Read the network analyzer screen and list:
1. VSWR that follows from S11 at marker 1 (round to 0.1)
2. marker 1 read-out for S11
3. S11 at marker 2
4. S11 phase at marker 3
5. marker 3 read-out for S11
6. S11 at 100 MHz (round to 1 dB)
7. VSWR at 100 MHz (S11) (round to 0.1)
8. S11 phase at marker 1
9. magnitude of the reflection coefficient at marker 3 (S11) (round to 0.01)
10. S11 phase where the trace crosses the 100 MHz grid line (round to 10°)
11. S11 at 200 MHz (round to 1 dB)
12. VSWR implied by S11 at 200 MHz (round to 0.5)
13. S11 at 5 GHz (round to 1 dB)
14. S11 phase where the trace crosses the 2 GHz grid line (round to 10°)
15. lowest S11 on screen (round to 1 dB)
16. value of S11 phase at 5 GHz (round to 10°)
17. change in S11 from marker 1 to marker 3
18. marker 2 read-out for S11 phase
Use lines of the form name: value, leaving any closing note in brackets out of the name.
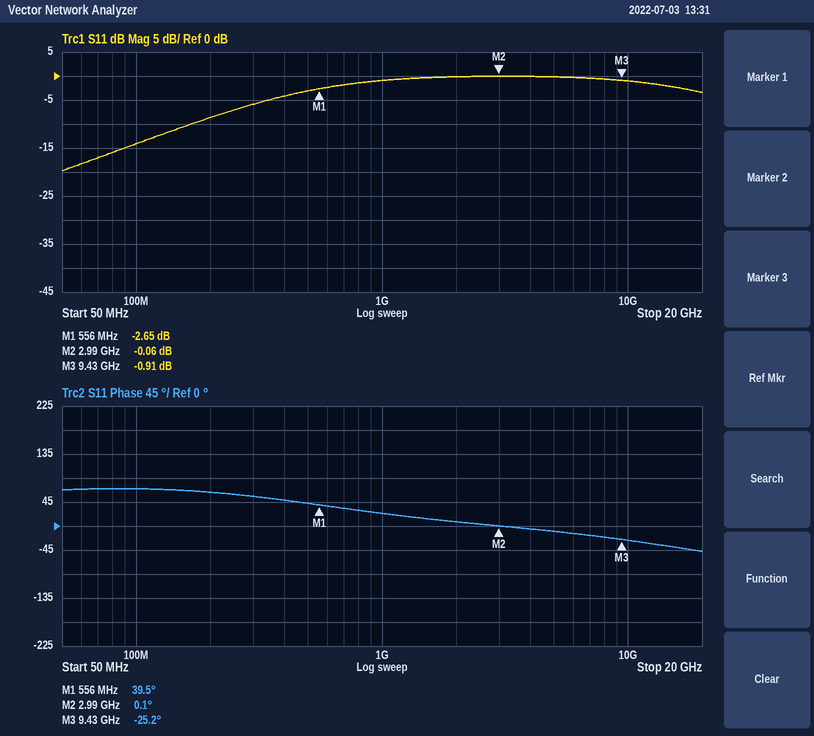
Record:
VSWR that follows from S11 at marker 1: 6.6
marker 1 read-out for S11: -2.65 dB
S11 at marker 2: -0.06 dB
S11 phase at marker 3: -25.2°
marker 3 read-out for S11: -0.91 dB
S11 at 100 MHz: -14 dB
VSWR at 100 MHz (S11): 1.5
S11 phase at marker 1: 39.5°
magnitude of the reflection coefficient at marker 3 (S11): 0.90
S11 phase where the trace crosses the 100 MHz grid line: 70°
S11 at 200 MHz: -9 dB
VSWR implied by S11 at 200 MHz: 2.0
S11 at 5 GHz: 0 dB
S11 phase where the trace crosses the 2 GHz grid line: 10°
lowest S11 on screen: -20 dB
value of S11 phase at 5 GHz: -10°
change in S11 from marker 1 to marker 3: 1.74 dB
marker 2 read-out for S11 phase: 0.1°
